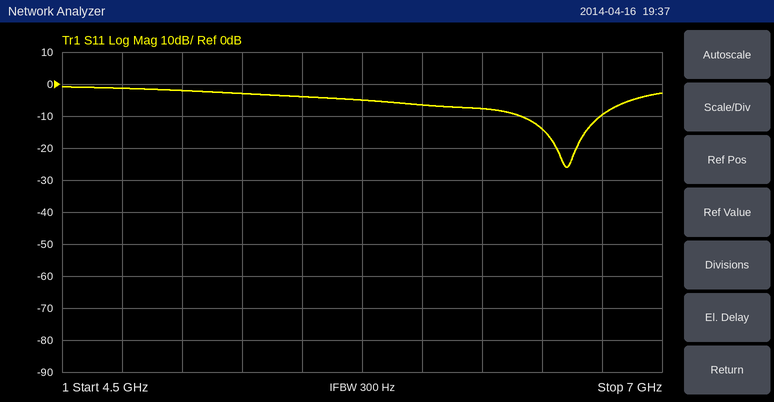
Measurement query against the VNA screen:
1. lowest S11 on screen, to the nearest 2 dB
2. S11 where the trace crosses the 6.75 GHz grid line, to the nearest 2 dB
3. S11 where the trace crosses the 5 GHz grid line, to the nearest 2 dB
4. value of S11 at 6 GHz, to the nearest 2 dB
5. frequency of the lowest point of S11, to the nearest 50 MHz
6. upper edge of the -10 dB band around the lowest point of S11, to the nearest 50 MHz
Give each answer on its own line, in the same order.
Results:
-26 dB
-10 dB
-2 dB
-6 dB
6.60 GHz
6.75 GHz
